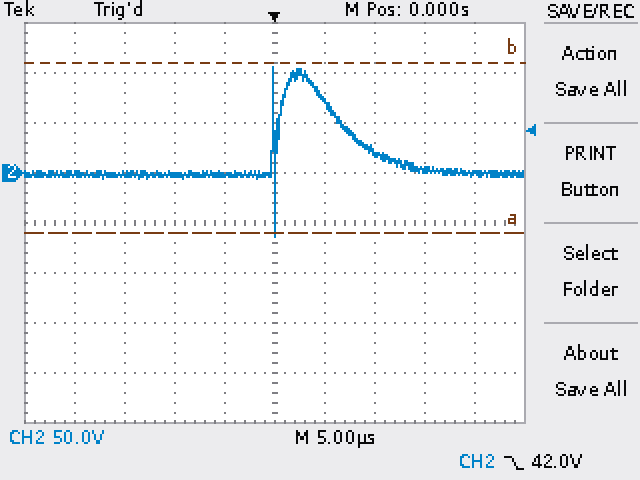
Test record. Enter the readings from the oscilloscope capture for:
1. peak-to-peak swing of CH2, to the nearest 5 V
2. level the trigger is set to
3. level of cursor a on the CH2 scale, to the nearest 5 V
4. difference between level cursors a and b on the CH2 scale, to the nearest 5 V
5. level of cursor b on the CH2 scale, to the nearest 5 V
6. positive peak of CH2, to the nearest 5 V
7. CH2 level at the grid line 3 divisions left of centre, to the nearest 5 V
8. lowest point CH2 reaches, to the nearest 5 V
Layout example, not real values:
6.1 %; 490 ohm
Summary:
170 V; 42.0 V; -60 V; 170 V; 110 V; 105 V; 0 V; -65 V
